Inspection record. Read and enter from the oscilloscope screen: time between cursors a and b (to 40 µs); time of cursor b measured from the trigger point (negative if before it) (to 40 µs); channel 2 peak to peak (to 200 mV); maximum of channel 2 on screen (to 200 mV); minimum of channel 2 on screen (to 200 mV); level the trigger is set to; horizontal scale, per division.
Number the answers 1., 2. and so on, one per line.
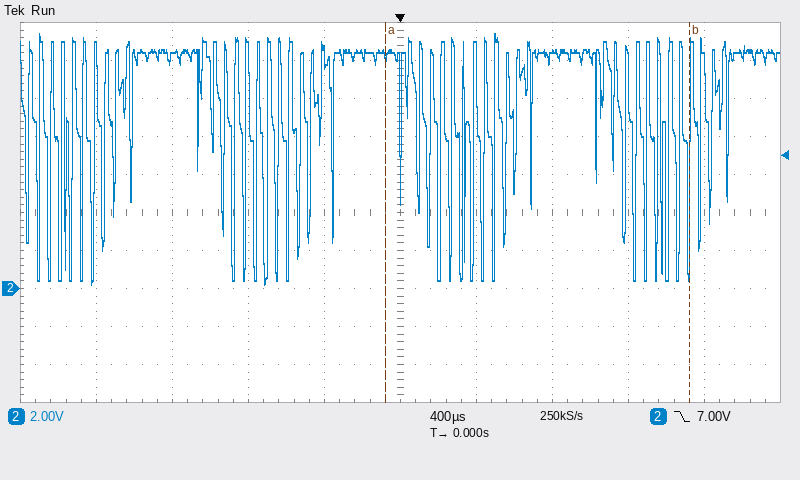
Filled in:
1. 1.60 ms
2. +1.52 ms
3. 13.2 V
4. 13.4 V
5. 200 mV
6. 7.00 V
7. 400 µs
